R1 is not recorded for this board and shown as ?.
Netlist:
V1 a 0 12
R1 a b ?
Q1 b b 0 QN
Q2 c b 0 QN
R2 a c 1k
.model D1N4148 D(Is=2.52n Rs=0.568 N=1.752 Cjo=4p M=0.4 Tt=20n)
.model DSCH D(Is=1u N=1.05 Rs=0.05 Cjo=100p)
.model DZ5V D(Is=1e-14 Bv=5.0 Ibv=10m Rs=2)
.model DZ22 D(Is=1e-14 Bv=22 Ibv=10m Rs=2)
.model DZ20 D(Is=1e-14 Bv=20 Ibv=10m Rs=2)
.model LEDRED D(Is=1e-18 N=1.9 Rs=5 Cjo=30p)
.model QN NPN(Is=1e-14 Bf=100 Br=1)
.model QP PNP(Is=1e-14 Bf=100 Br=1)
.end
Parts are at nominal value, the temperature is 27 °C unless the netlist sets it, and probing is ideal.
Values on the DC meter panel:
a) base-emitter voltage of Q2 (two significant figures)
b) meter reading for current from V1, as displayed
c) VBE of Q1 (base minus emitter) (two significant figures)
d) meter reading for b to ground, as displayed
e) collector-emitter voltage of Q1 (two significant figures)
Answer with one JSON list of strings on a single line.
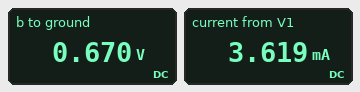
["670 mV", "3.619 mA", "670 mV", "0.670 V", "670 mV"]
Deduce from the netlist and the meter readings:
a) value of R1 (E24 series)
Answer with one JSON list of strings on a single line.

["6.2 kΩ"]
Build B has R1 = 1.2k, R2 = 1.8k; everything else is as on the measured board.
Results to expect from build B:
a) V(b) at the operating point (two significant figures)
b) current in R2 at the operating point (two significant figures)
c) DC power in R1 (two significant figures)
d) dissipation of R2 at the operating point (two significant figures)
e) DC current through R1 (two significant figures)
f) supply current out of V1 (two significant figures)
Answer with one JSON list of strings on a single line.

["710 mV", "6.6 mA", "110 mW", "79 mW", "9.4 mA", "16 mA"]
